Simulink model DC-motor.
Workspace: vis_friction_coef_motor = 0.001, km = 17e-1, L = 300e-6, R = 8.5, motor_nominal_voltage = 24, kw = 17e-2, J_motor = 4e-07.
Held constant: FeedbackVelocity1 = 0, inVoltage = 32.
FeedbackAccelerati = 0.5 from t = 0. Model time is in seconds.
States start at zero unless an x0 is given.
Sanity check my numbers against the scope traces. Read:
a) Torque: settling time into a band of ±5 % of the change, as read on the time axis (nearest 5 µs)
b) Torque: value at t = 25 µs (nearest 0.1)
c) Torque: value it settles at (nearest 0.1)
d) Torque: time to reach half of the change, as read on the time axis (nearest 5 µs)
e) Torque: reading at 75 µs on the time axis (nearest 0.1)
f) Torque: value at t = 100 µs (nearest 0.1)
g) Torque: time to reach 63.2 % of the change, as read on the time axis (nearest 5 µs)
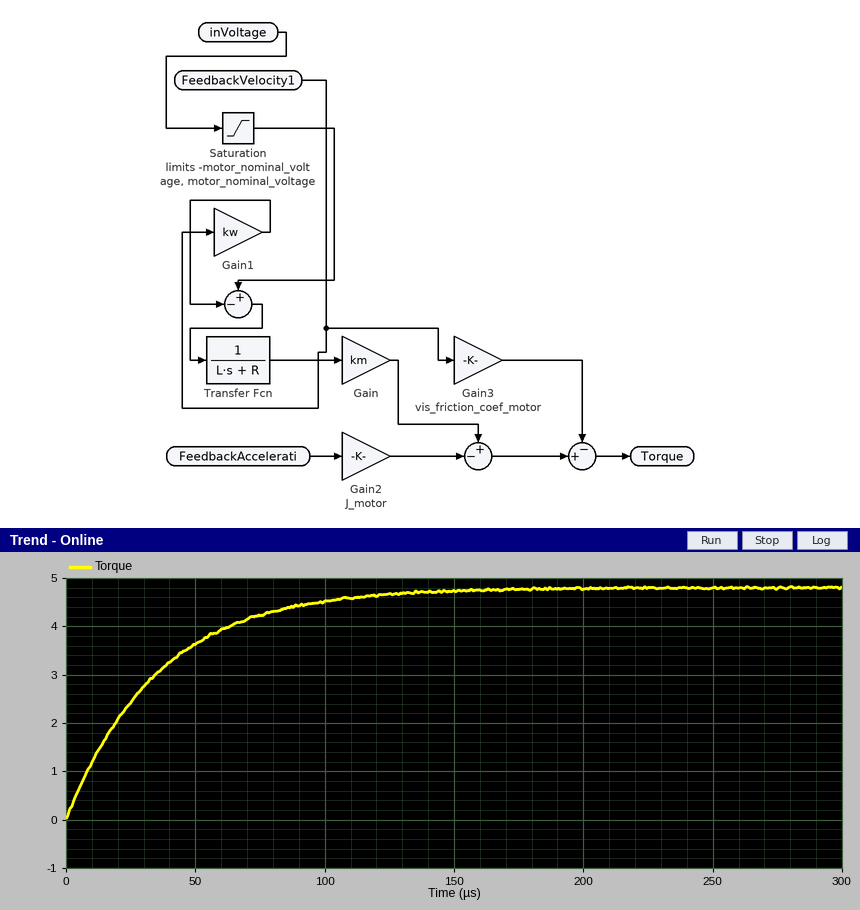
105 µs
2.4
4.8
25 µs
4.2
4.5
35 µs
